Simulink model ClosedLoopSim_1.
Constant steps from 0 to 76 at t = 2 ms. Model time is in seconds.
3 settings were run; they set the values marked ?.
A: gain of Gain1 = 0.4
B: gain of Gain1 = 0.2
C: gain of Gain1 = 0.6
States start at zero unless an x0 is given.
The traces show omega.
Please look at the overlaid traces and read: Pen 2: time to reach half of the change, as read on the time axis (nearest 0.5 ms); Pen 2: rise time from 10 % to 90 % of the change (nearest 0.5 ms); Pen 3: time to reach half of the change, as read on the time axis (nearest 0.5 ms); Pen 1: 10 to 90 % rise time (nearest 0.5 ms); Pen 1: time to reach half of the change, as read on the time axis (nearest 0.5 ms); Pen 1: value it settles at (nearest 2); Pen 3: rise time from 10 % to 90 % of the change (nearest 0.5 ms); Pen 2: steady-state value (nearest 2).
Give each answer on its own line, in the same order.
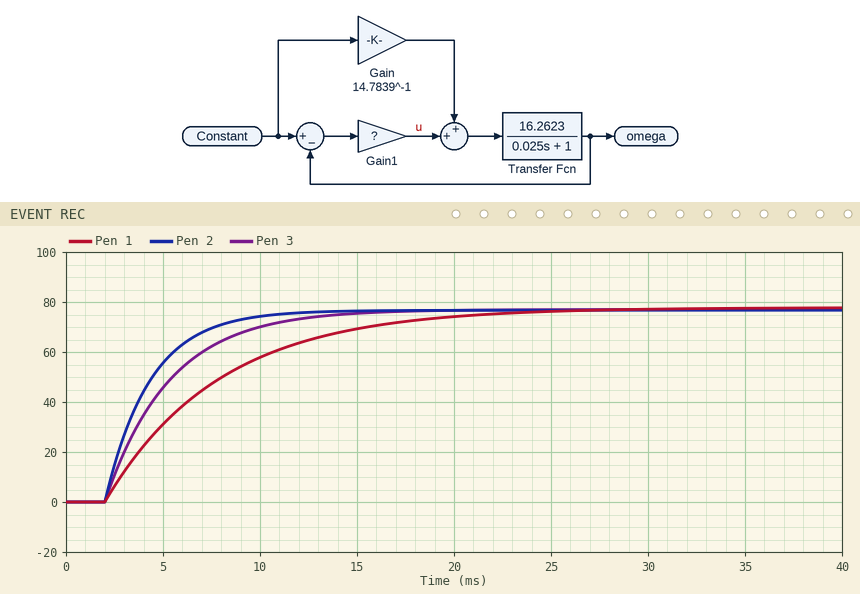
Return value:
3.5 ms
5.0 ms
4.5 ms
13.0 ms
6.0 ms
78
7.5 ms
76
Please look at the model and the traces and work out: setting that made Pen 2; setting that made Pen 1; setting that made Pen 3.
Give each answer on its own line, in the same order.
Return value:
C
B
A
